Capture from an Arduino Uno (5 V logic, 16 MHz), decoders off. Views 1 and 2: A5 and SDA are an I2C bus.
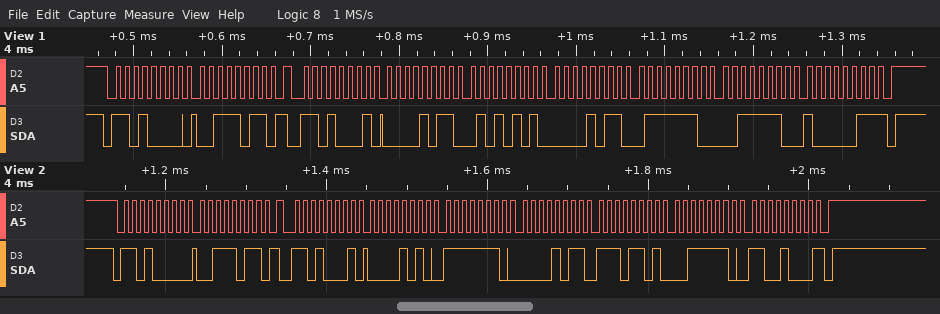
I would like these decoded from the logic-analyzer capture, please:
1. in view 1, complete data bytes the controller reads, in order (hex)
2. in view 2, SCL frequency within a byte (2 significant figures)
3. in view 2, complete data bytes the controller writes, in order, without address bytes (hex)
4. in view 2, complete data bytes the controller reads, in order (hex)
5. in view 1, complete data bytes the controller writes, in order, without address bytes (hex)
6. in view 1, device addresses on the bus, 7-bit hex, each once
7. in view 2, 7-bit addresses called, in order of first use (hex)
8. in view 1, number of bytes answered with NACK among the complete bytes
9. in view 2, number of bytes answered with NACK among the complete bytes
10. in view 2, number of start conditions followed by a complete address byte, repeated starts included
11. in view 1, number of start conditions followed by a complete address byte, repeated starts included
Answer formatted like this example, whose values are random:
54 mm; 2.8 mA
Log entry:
0B 55 0B 7E 3E 83; 100 kHz; 3B; 0A FE 0B ED 3E C8; 3B; 0x68; 0x68; 1; 1; 2; 2
